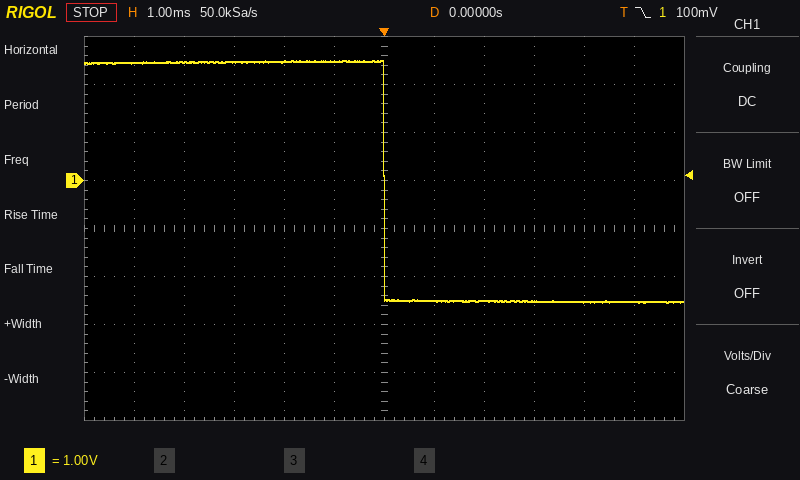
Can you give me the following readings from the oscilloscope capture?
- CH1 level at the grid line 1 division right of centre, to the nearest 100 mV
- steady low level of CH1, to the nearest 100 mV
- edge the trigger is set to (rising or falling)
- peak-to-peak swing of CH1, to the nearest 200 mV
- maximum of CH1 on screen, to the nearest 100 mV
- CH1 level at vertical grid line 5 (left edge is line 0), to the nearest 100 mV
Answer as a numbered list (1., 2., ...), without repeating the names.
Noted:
1. -2.5 V
2. -2.5 V
3. falling
4. 5.0 V
5. 2.5 V
6. 2.5 V
